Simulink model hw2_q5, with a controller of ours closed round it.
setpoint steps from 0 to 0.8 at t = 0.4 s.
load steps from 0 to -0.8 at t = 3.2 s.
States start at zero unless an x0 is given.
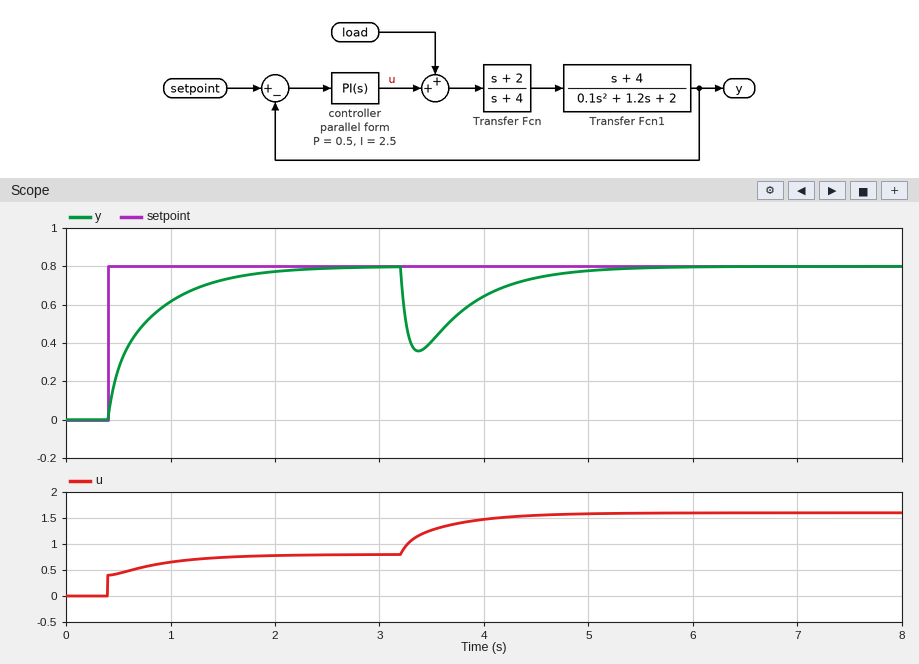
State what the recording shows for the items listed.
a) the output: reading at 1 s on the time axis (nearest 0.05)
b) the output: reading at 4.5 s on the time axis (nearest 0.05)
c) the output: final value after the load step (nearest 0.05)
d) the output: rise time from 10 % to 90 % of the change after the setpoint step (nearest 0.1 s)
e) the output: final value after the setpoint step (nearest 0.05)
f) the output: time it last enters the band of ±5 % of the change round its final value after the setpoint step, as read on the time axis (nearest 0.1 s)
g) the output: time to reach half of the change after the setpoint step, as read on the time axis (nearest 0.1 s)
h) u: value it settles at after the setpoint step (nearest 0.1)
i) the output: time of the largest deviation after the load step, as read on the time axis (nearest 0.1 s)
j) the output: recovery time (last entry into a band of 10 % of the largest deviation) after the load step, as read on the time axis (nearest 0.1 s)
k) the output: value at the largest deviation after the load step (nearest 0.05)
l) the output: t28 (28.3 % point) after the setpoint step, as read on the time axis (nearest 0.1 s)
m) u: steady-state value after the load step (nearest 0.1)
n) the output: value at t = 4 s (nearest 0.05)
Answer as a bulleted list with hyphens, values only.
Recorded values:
- 0.60
- 0.75
- 0.80
- 1.0 s
- 0.80
- 1.8 s
- 0.6 s
- 0.8
- 3.4 s
- 4.7 s
- 0.35
- 0.5 s
- 1.6
- 0.65
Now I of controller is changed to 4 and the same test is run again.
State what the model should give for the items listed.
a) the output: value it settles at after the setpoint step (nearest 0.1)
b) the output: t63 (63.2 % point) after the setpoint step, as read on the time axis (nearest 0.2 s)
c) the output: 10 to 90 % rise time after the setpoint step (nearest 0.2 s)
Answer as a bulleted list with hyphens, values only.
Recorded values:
- 0.8
- 0.6 s
- 0.6 s
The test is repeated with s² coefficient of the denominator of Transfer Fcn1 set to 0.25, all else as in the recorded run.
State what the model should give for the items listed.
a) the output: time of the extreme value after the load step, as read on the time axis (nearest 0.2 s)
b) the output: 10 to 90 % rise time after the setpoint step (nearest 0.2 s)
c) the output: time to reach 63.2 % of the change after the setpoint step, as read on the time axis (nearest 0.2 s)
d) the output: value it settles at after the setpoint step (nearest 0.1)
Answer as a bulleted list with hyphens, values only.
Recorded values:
- 3.6 s
- 0.8 s
- 0.8 s
- 0.8
